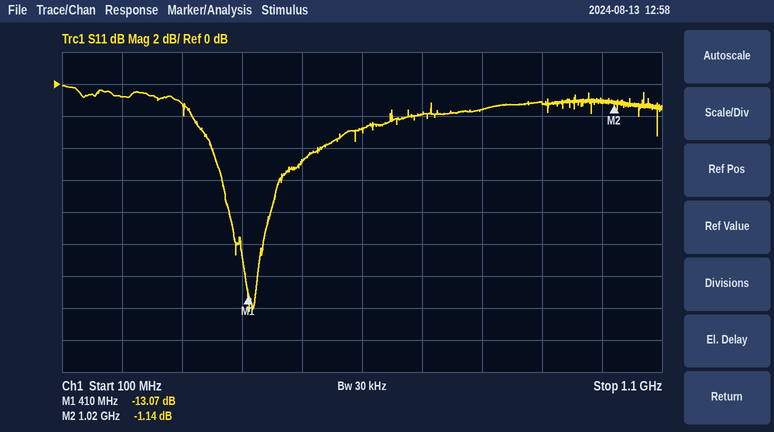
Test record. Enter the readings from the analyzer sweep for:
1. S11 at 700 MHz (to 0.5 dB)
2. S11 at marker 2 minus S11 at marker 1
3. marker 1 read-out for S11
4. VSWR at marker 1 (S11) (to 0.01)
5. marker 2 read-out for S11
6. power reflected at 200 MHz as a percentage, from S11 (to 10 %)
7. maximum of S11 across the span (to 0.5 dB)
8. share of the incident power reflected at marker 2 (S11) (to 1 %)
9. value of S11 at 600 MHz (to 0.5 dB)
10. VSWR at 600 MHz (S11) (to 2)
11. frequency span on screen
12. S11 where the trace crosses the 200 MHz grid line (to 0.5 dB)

-2.0 dB
11.93 dB
-13.07 dB
1.57
-1.14 dB
80 %
0.0 dB
77 %
-3.0 dB
6
1 GHz
-1.0 dB
